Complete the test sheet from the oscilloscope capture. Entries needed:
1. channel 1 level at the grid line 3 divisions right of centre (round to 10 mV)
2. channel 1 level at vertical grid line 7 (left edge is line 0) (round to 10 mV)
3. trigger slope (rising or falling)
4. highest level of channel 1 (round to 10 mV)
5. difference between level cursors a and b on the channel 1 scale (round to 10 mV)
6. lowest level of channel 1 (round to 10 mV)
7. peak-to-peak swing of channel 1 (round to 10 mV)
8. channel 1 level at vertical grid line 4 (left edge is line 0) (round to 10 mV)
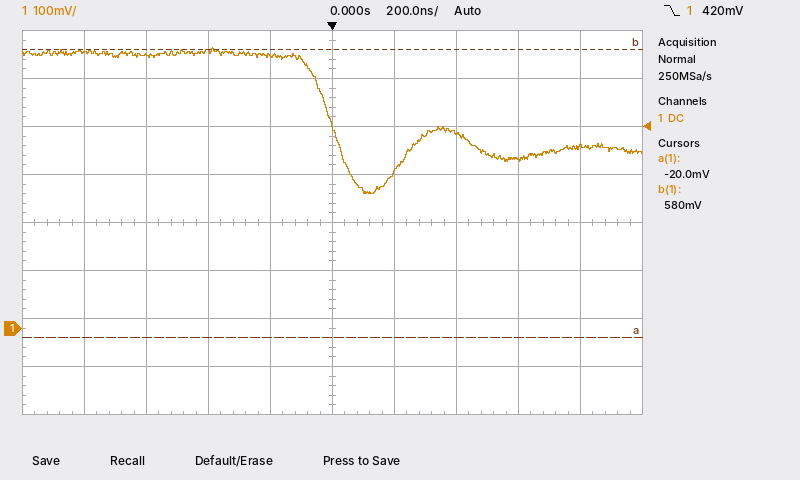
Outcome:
350 mV
410 mV
falling
580 mV
600 mV
280 mV
300 mV
570 mV
